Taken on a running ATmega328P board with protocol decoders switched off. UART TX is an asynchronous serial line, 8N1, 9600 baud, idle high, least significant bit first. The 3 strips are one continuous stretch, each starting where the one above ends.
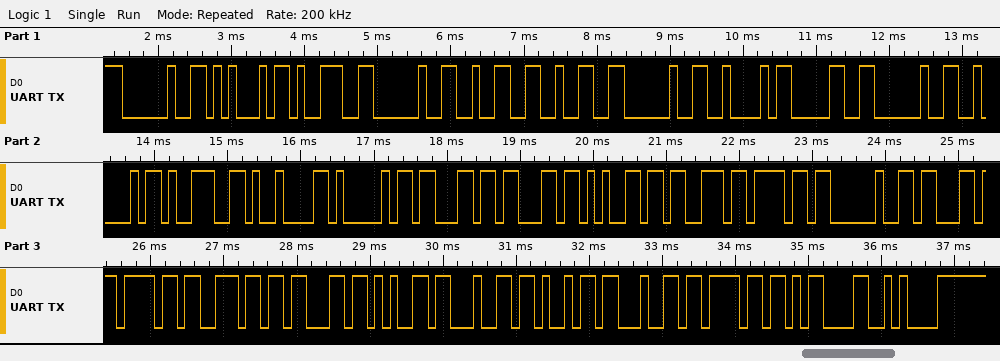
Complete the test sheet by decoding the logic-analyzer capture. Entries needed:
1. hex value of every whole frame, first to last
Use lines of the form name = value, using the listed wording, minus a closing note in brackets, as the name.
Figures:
hex value of every whole frame, first to last = 0x20 0x45 0x39 0x20 0x32 0x32 0x20 0x42 0x30 0x20 0x42 0x39 0x09 0x41 0x63 0x63 0x65 0x73 0x6F 0x20 0x63 0x6F 0x6E 0x63 0x65 0x64 0x69 0x64 0x6F 0x0D 0x0A
